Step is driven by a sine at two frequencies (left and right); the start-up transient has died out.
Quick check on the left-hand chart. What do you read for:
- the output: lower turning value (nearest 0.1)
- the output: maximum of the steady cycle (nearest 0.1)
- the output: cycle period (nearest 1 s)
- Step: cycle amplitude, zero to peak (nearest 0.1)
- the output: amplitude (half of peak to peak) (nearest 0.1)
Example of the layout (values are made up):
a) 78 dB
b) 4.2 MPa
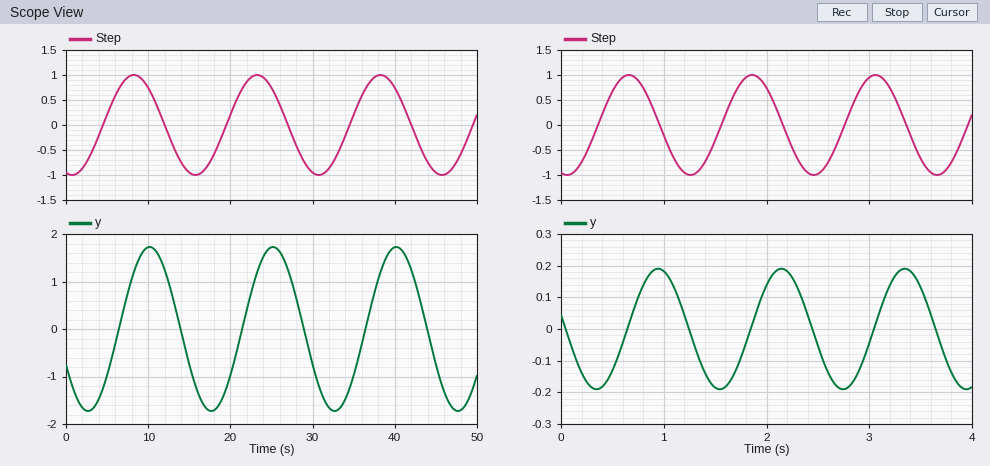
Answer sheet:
a) -1.7
b) 1.7
c) 15 s
d) 1.0
e) 1.7
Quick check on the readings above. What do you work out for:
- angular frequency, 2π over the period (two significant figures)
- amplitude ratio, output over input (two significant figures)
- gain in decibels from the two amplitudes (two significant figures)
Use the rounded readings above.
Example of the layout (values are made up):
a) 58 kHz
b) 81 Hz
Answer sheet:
a) 0.42 rad/s
b) 1.7
c) 4.6 dB
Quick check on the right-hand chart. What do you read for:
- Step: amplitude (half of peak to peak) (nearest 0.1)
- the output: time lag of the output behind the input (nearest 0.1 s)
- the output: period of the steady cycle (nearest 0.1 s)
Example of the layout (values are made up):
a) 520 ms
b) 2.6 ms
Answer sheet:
a) 1.0
b) 0.3 s
c) 1.2 s
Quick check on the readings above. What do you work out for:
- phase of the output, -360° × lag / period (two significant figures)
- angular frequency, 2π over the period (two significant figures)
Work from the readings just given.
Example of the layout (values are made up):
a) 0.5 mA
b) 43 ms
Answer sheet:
a) -90°
b) 5.2 rad/s
